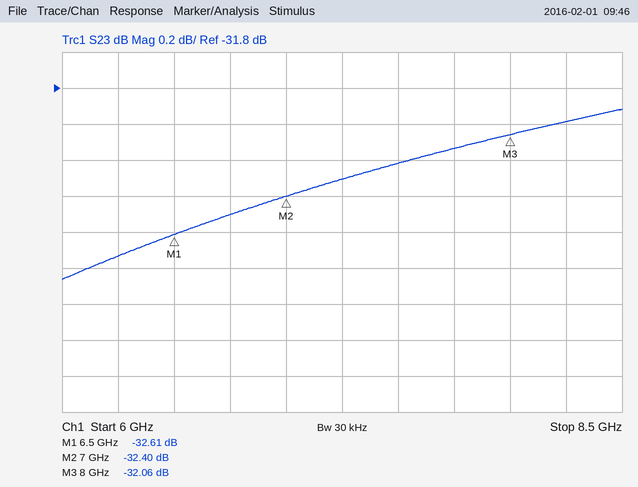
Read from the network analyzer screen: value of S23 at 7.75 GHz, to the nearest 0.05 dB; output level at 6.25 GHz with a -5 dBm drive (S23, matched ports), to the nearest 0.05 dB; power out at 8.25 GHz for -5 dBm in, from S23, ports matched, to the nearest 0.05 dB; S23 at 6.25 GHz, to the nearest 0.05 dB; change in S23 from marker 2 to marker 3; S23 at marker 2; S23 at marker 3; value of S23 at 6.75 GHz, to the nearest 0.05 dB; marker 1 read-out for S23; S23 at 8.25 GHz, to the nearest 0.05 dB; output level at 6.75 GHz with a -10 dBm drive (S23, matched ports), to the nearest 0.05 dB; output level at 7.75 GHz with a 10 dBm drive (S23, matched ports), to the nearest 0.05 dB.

-32.15 dB
-37.75 dBm
-37.00 dBm
-32.75 dB
0.34 dB
-32.40 dB
-32.06 dB
-32.50 dB
-32.61 dB
-32.00 dB
-42.50 dBm
-22.15 dBm
